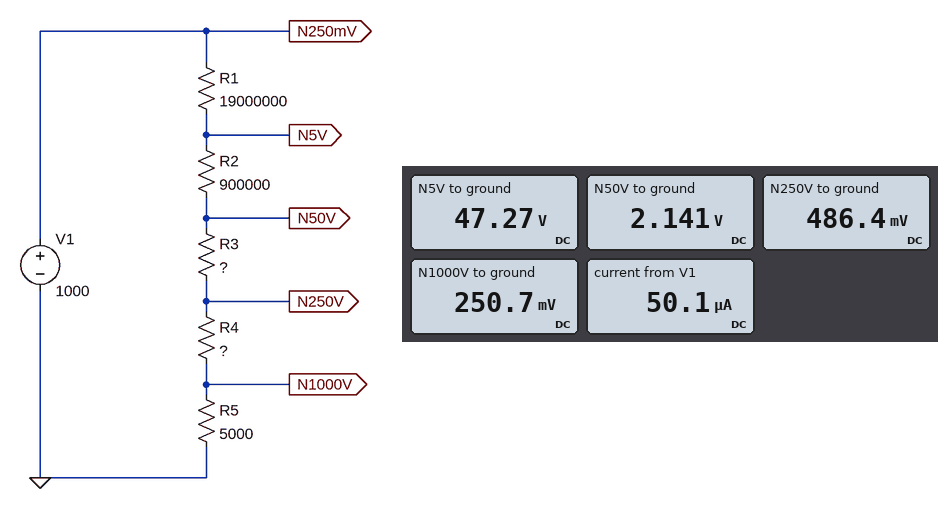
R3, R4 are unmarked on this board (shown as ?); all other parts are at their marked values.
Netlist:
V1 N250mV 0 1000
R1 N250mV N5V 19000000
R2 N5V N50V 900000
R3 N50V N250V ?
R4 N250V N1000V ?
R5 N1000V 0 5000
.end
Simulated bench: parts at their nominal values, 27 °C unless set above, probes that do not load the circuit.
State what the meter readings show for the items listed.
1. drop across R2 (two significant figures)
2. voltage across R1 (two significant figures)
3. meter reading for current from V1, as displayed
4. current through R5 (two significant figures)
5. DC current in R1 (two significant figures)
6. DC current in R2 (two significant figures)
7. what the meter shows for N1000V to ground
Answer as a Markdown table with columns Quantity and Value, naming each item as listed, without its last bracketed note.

| Quantity | Value |
|---|---|
| drop across R2 | 45 V |
| voltage across R1 | 950 V |
| meter reading for current from V1, as displayed | 50.1 µA |
| current through R5 | 50 µA |
| DC current in R1 | 50 µA |
| DC current in R2 | 50 µA |
| what the meter shows for N1000V to ground | 250.7 mV |
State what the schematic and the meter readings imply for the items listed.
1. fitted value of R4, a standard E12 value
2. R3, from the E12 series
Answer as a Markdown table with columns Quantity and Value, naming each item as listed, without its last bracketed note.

| Quantity | Value |
|---|---|
| fitted value of R4, a standard E12 value | 4.7 kΩ |
| R3, from the E12 series | 33 kΩ |
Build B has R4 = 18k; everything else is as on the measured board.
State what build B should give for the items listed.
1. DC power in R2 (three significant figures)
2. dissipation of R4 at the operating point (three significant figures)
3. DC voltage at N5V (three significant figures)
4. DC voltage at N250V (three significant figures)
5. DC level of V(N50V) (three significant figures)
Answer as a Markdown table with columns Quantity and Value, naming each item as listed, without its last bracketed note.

| Quantity | Value |
|---|---|
| DC power in R2 | 2.26 mW |
| dissipation of R4 at the operating point | 45.2 µW |
| DC voltage at N5V | 47.9 V |
| DC voltage at N250V | 1.15 V |
| DC level of V(N50V) | 2.81 V |
